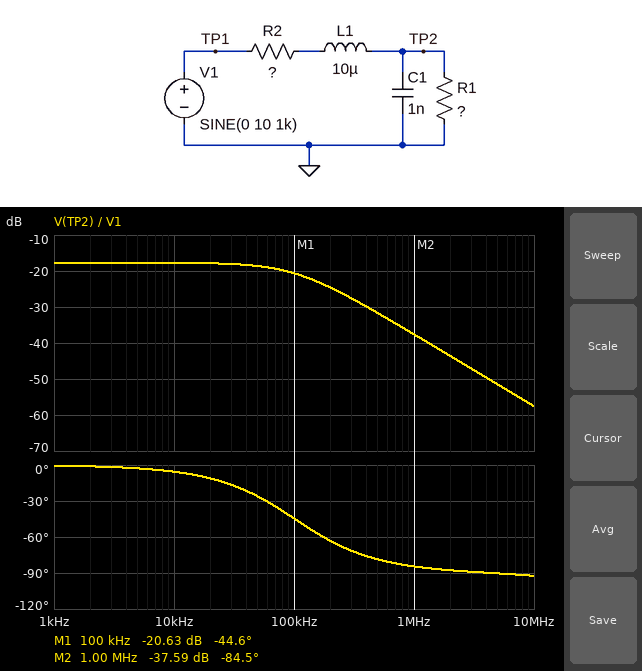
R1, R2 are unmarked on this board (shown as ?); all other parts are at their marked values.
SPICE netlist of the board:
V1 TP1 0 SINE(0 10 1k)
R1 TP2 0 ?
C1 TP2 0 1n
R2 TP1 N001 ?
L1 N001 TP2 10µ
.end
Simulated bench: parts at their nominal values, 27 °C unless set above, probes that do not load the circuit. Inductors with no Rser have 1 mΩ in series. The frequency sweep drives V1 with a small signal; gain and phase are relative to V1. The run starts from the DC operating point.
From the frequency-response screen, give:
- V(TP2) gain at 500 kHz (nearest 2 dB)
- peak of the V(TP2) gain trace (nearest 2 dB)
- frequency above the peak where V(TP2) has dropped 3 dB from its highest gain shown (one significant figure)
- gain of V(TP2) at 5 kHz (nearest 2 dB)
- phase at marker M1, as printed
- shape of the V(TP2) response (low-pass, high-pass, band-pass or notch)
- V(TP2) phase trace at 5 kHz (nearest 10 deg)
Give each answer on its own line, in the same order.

-32 dB
-18 dB
100 kHz
-18 dB
-44.6 deg
low-pass
0 deg
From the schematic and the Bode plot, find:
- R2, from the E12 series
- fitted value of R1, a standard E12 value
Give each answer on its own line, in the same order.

12 kΩ
1.8 kΩ
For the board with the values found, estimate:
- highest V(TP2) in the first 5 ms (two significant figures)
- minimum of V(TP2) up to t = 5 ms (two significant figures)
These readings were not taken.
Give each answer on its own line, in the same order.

1.3 V
-1.3 V
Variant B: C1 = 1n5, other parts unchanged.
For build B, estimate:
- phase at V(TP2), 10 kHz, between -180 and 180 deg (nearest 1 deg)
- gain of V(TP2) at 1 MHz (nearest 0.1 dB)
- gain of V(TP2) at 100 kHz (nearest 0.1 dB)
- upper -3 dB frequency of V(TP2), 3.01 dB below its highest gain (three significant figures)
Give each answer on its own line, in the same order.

-8 deg
-41.1 dB
-22.7 dB
67.8 kHz
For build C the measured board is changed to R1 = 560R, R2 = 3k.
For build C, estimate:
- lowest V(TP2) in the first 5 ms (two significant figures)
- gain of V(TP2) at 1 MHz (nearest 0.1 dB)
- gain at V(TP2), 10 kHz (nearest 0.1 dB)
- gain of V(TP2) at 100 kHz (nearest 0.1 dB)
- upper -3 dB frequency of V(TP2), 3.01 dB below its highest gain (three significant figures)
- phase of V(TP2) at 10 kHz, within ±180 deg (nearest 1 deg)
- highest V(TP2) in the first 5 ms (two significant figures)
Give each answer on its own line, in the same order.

-1.6 V
-26.0 dB
-16.1 dB
-16.4 dB
338 kHz
-2 deg
1.6 V
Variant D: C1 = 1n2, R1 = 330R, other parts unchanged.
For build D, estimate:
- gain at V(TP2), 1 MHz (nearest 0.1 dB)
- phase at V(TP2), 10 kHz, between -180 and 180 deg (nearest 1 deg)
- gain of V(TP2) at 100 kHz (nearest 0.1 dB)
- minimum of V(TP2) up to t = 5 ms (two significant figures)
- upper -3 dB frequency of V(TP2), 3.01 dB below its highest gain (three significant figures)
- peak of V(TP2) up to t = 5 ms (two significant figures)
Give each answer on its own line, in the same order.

-39.8 dB
-1 deg
-31.7 dB
-270 mV
413 kHz
270 mV
